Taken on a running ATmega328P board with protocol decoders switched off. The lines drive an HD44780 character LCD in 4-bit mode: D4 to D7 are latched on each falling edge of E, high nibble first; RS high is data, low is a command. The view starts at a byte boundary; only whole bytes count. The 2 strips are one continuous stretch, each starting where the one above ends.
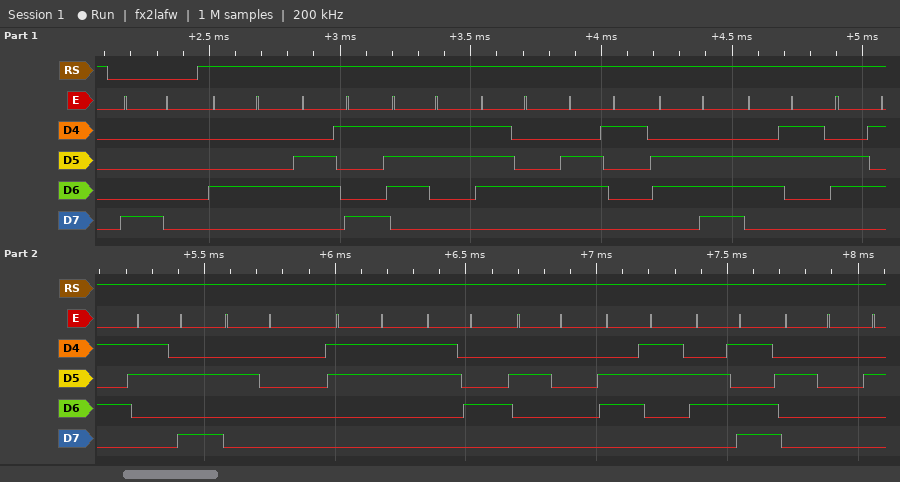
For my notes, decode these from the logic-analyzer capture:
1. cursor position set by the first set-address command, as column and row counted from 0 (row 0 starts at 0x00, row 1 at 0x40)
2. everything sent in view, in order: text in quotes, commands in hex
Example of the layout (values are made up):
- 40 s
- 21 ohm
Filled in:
- column 0, row 0
- 0x80 "Distance: 34 cm "
